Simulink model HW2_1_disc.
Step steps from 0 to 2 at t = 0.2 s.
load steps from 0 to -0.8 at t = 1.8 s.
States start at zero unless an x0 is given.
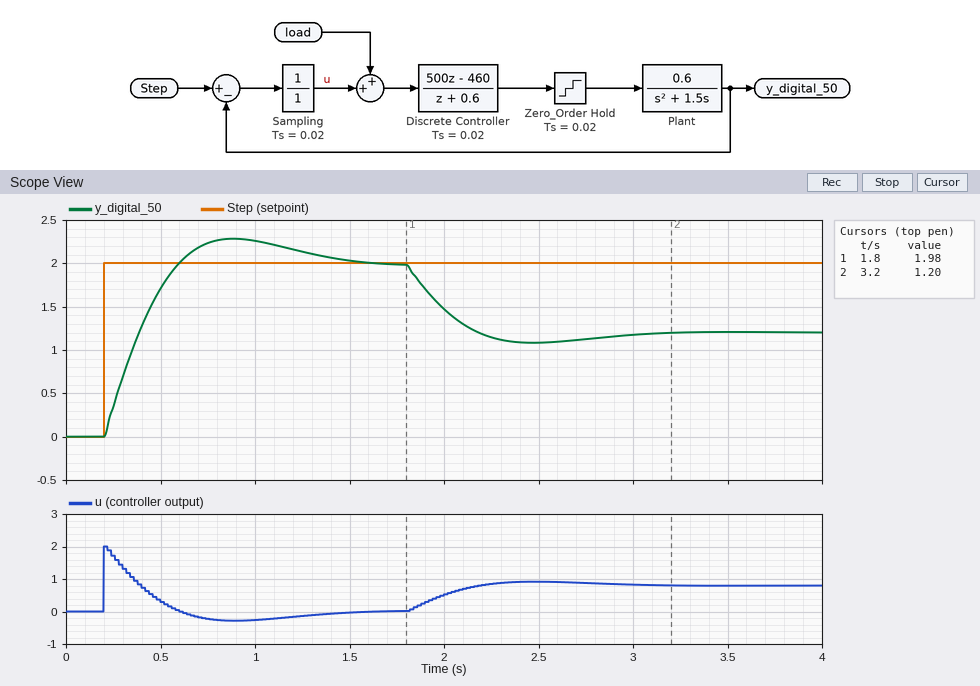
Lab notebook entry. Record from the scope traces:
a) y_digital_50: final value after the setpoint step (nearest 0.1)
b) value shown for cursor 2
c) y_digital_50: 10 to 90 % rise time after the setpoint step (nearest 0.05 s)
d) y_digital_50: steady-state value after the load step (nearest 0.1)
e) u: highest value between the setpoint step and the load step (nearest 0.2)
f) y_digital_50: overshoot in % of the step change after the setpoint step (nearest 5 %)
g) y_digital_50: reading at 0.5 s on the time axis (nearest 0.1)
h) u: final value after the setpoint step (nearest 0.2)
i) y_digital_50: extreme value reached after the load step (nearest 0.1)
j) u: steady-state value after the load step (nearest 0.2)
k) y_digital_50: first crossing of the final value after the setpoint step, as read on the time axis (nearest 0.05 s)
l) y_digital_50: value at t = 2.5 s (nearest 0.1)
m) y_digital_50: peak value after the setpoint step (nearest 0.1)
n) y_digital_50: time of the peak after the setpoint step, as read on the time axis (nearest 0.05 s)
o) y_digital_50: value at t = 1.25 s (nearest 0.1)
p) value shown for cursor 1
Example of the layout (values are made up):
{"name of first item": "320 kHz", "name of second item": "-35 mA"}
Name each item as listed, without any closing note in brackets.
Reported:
{"y_digital_50: final value after the setpoint step": "2.0", "value shown for cursor 2": "1.20", "y_digital_50: 10 to 90 % rise time after the setpoint step": "0.30 s", "y_digital_50: steady-state value after the load step": "1.2", "u: highest value between the setpoint step and the load step": "2.0", "y_digital_50: overshoot in % of the step change after the setpoint step": "15 %", "y_digital_50: reading at 0.5 s on the time axis": "1.7", "u: final value after the setpoint step": "0.0", "y_digital_50: extreme value reached after the load step": "1.1", "u: steady-state value after the load step": "0.8", "y_digital_50: first crossing of the final value after the setpoint step, as read on the time axis": "0.60 s", "y_digital_50: value at t = 2.5 s": "1.1", "y_digital_50: peak value after the setpoint step": "2.3", "y_digital_50: time of the peak after the setpoint step, as read on the time axis": "0.90 s", "y_digital_50: value at t = 1.25 s": "2.1", "value shown for cursor 1": "1.98"}
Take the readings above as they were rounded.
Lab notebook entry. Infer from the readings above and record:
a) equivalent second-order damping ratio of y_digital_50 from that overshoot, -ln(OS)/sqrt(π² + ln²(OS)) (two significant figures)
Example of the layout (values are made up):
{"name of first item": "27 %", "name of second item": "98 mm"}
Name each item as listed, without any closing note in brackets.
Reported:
{"equivalent second-order damping ratio of y_digital_50 from that overshoot, -ln(OS)/sqrt(π² + ln²(OS))": "0.52"}
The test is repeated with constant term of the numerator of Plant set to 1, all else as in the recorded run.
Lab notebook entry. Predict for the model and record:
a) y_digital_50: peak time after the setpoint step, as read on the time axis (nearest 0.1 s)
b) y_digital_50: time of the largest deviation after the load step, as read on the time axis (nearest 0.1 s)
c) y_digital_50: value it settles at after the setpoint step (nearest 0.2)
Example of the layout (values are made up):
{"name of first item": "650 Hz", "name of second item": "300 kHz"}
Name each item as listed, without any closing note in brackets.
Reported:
{"y_digital_50: peak time after the setpoint step, as read on the time axis": "0.7 s", "y_digital_50: time of the largest deviation after the load step, as read on the time axis": "2.3 s", "y_digital_50: value it settles at after the setpoint step": "2.0"}
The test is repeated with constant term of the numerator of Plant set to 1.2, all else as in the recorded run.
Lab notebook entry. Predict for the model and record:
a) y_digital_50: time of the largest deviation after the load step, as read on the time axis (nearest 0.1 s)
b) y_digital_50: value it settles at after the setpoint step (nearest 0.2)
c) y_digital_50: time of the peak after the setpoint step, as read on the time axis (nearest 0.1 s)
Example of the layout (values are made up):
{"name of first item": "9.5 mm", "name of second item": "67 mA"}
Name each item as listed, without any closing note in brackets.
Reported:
{"y_digital_50: time of the largest deviation after the load step, as read on the time axis": "2.2 s", "y_digital_50: value it settles at after the setpoint step": "2.0", "y_digital_50: time of the peak after the setpoint step, as read on the time axis": "0.6 s"}
